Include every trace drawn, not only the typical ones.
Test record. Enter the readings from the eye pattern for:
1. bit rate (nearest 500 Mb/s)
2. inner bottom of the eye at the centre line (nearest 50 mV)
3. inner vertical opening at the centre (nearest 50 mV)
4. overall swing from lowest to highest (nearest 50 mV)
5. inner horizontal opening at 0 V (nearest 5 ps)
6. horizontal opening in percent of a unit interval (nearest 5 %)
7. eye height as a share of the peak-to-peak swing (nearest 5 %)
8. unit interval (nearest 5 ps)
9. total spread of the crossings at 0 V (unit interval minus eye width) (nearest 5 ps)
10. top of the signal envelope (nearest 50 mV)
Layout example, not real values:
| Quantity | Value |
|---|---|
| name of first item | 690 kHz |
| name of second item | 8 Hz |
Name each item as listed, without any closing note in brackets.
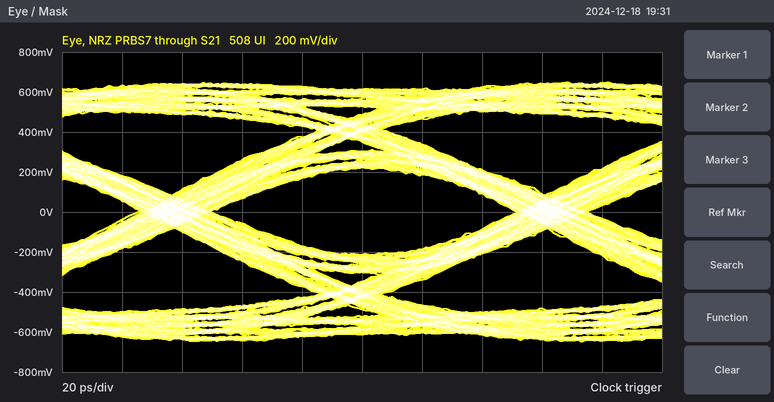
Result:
| Quantity | Value |
|---|---|
| bit rate | 8.0 Gb/s |
| inner bottom of the eye at the centre line | -200 mV |
| inner vertical opening at the centre | 450 mV |
| overall swing from lowest to highest | 1.30 V |
| inner horizontal opening at 0 V | 100 ps |
| horizontal opening in percent of a unit interval | 80 % |
| eye height as a share of the peak-to-peak swing | 35 % |
| unit interval | 125 ps |
| total spread of the crossings at 0 V (unit interval minus eye width) | 25 ps |
| top of the signal envelope | 650 mV |
